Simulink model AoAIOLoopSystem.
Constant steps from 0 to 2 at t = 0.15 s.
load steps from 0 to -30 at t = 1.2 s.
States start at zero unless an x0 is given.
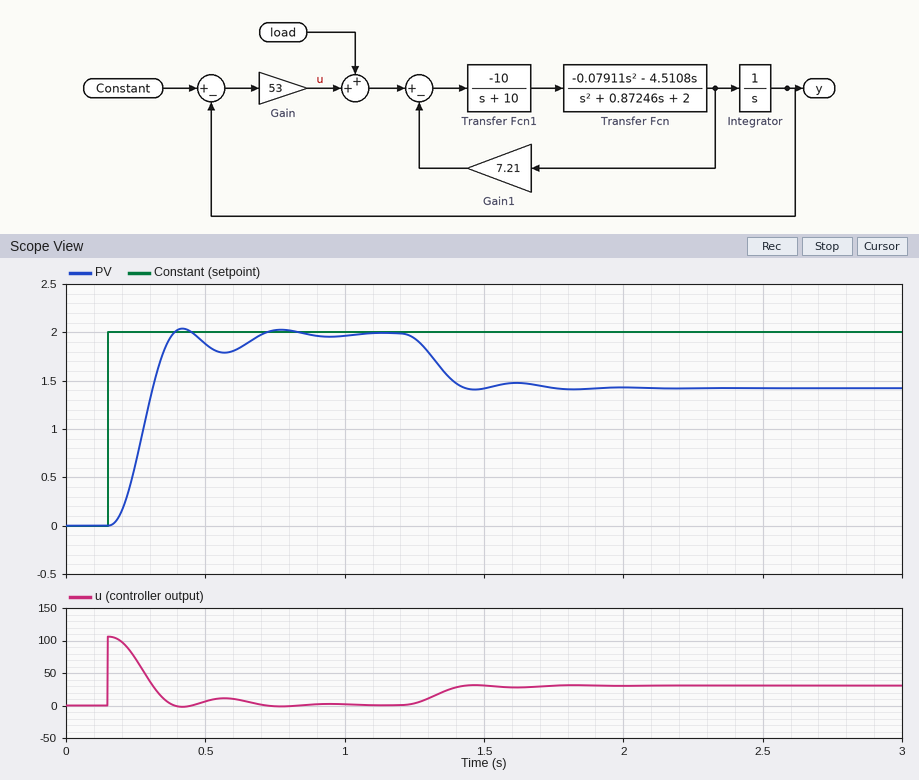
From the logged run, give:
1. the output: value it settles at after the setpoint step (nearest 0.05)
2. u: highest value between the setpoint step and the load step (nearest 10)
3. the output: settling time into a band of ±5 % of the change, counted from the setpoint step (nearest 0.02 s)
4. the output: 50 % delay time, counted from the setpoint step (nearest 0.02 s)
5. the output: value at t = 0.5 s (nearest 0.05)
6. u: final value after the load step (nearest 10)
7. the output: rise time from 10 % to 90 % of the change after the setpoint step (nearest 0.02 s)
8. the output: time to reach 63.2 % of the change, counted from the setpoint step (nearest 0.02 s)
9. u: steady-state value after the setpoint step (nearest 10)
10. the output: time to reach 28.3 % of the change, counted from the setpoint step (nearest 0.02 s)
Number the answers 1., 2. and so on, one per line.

1. 2.00
2. 110
3. 0.50 s
4. 0.12 s
5. 1.90
6. 30
7. 0.14 s
8. 0.14 s
9. 0
10. 0.10 s
